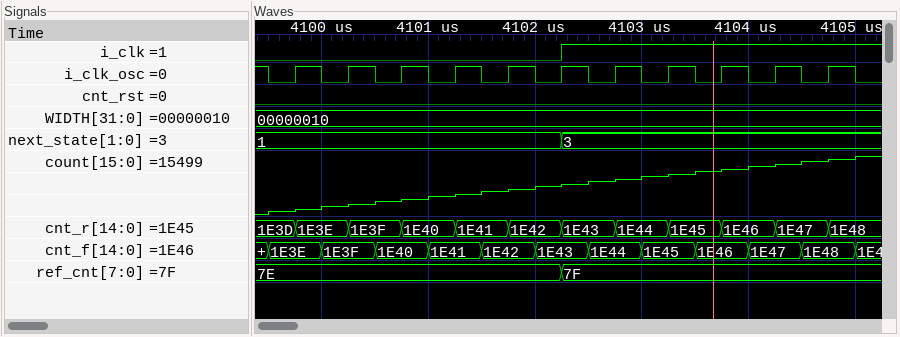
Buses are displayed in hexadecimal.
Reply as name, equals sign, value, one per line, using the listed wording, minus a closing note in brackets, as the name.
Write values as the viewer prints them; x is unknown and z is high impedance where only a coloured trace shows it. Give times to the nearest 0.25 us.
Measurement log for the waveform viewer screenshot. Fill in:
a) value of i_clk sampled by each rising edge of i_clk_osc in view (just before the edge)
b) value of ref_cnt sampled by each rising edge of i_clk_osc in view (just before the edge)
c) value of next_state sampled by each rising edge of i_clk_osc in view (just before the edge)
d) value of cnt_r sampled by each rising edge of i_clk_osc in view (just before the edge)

value of i_clk sampled by each rising edge of i_clk_osc in view = 0 0 0 0 0 0 1 1 1 1 1
value of ref_cnt sampled by each rising edge of i_clk_osc in view = 7E, 7E, 7E, 7E, 7E, 7E, 7F, 7F, 7F, 7F, 7F
value of next_state sampled by each rising edge of i_clk_osc in view = 1, 1, 1, 1, 1, 1, 3, 3, 3, 3, 3
value of cnt_r sampled by each rising edge of i_clk_osc in view = 1E3D, 1E3E, 1E3F, 1E40, 1E41, 1E42, 1E43, 1E44, 1E45, 1E46, 1E47
